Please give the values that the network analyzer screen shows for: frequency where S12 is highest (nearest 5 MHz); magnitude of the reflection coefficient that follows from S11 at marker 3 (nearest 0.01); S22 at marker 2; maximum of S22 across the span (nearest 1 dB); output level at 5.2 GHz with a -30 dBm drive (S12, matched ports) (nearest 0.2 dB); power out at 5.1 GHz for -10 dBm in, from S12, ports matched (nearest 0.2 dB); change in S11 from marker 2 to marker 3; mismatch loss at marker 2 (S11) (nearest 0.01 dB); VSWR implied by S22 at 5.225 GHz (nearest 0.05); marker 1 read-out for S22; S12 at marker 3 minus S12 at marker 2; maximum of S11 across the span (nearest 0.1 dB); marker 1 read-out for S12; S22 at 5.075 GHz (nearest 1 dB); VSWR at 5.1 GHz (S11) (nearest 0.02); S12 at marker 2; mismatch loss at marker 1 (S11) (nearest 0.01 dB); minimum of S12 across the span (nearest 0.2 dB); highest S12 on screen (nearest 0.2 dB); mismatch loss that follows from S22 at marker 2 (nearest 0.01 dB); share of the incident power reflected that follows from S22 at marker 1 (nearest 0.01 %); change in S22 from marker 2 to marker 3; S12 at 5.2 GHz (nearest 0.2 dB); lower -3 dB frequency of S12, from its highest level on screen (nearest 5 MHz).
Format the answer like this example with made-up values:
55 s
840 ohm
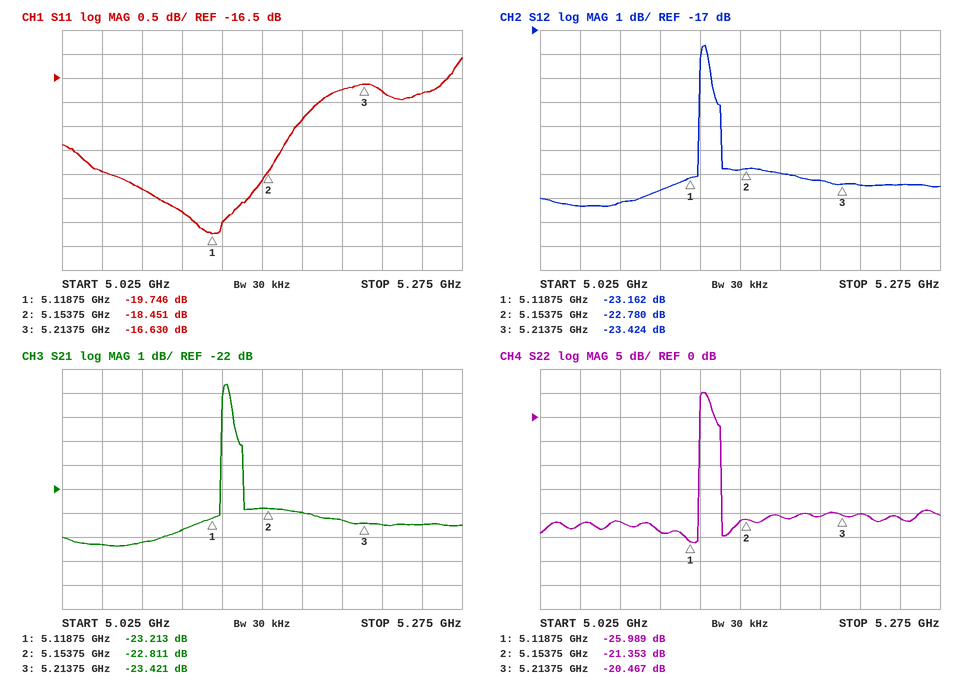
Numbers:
5.130 GHz
0.15
-21.353 dB
5 dB
-53.2 dBm
-33.6 dBm
1.821 dB
0.06 dB
1.20
-25.989 dB
-0.644 dB
-16.1 dB
-23.162 dB
-22 dB
1.24
-22.780 dB
0.05 dB
-24.4 dB
-17.6 dB
0.03 dB
0.25 %
0.886 dB
-23.2 dB
5.125 GHz
